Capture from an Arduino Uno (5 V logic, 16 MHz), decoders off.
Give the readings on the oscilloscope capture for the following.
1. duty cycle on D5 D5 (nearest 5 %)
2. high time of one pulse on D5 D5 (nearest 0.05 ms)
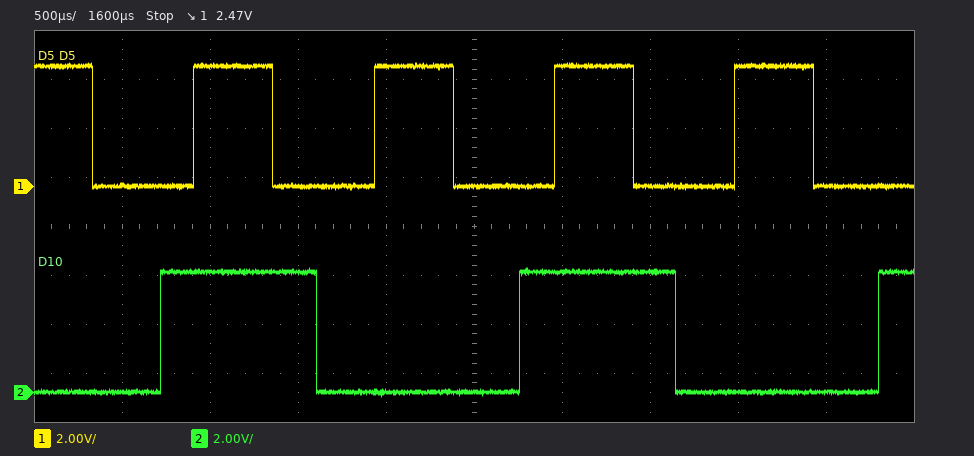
45 %
0.45 ms
